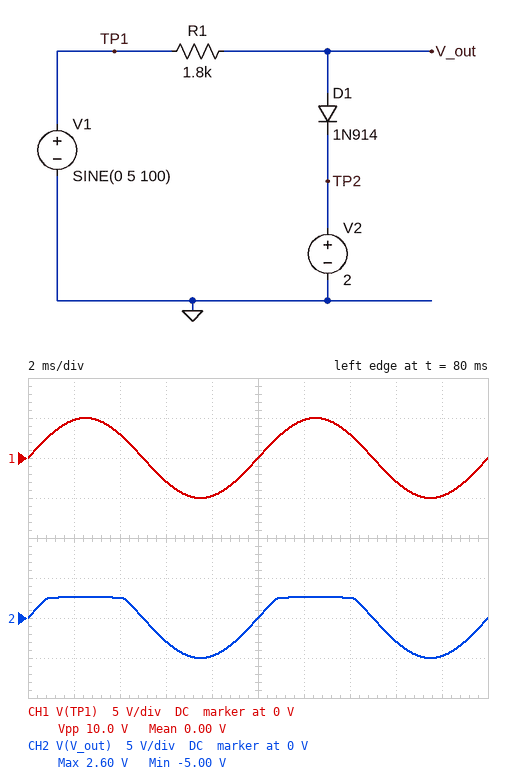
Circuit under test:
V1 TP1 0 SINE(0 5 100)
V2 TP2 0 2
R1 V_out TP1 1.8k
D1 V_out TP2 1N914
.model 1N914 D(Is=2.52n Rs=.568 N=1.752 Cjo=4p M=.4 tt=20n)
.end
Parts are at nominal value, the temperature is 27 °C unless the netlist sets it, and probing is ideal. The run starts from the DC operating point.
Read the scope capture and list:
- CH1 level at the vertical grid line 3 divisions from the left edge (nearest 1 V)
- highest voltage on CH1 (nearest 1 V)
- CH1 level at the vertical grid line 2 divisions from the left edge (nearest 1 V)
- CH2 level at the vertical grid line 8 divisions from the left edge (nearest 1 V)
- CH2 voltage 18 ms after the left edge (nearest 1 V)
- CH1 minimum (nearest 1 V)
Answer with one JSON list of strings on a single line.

["-3 V", "5 V", "3 V", "-3 V", "-5 V", "-5 V"]
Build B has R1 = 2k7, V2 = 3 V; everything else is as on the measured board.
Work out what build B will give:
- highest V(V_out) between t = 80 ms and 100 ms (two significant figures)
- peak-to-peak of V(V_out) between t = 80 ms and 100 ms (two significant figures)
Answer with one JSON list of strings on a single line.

["3.6 V", "8.6 V"]
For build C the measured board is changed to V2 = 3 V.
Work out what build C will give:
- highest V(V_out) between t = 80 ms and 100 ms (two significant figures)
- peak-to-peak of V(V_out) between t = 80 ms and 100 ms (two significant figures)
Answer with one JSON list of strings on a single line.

["3.6 V", "8.6 V"]
